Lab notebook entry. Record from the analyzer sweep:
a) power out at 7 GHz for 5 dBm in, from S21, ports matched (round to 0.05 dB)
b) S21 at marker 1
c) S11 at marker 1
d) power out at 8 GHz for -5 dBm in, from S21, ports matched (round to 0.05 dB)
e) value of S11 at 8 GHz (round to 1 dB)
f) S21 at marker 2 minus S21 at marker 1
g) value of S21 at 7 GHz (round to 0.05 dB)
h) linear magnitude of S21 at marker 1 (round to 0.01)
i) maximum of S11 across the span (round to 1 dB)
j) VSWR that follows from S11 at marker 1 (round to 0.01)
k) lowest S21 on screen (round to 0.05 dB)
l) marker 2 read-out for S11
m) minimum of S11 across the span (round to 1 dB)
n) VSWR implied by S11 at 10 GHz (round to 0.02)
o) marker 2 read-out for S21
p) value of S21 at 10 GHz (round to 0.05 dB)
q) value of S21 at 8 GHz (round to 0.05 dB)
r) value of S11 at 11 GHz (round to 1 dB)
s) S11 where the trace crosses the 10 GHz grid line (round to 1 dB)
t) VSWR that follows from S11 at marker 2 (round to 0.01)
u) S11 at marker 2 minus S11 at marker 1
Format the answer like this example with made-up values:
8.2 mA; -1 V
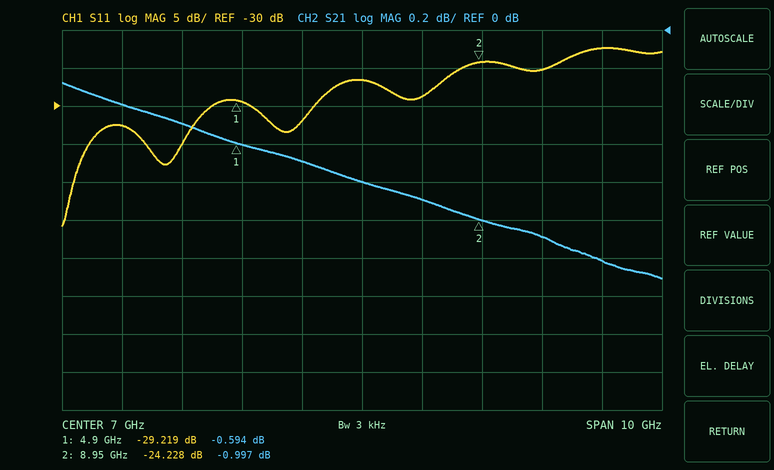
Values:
4.20 dBm; -0.594 dB; -29.219 dB; -5.90 dBm; -29 dB; -0.403 dB; -0.80 dB; 0.93; -22 dB; 1.07; -1.30 dB; -24.228 dB; -46 dB; 1.12; -0.997 dB; -1.10 dB; -0.90 dB; -22 dB; -25 dB; 1.13; 4.991 dB
